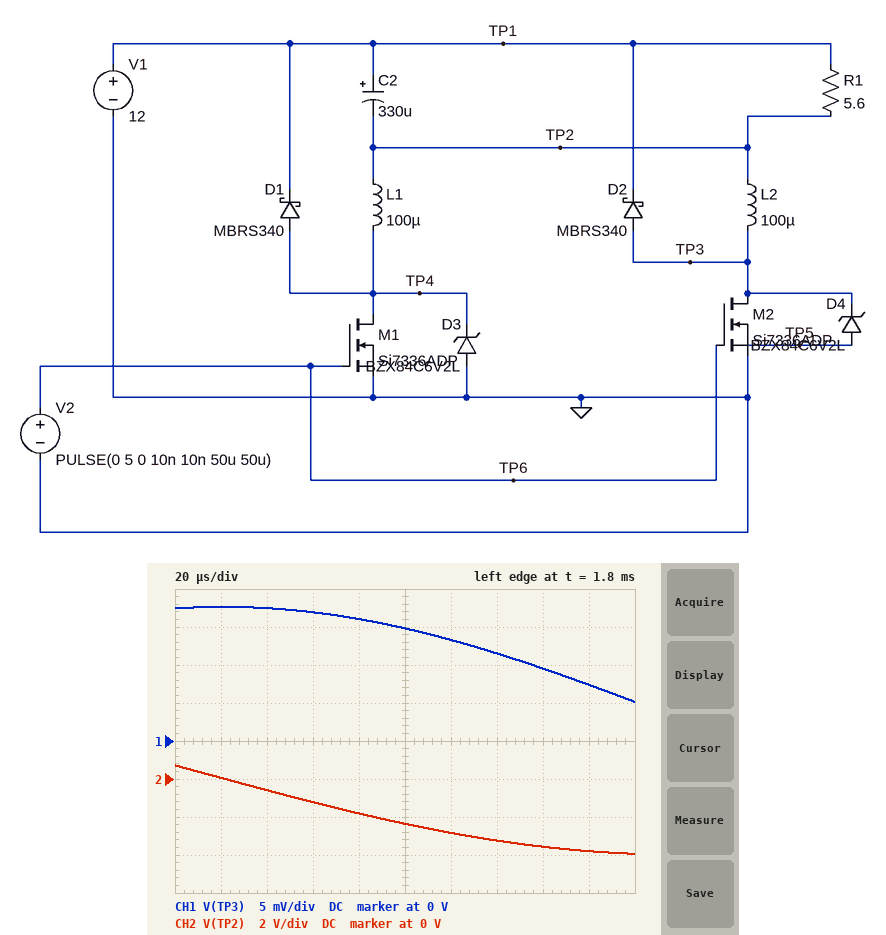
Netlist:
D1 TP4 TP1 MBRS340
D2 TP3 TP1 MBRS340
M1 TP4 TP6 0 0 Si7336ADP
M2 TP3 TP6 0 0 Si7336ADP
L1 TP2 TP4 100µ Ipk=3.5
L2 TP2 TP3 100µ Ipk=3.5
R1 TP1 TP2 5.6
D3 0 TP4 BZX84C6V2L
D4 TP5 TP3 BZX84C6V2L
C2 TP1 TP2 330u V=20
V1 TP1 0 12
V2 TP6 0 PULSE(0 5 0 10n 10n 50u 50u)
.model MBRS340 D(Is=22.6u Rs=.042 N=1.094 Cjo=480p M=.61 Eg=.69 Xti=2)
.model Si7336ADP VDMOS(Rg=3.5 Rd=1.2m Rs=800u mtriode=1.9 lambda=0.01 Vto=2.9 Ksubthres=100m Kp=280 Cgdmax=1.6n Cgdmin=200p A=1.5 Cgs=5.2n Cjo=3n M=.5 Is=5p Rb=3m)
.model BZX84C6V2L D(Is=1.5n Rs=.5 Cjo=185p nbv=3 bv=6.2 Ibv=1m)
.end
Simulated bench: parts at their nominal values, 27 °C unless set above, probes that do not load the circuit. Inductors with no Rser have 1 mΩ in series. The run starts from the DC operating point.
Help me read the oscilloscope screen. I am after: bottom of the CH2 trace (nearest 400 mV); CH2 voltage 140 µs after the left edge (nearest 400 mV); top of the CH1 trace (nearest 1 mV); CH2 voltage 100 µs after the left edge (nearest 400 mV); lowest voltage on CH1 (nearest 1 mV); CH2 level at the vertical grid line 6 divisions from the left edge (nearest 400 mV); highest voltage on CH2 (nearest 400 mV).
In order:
-4.0 V
-3.2 V
18 mV
-2.4 V
5 mV
-2.8 V
800 mV
